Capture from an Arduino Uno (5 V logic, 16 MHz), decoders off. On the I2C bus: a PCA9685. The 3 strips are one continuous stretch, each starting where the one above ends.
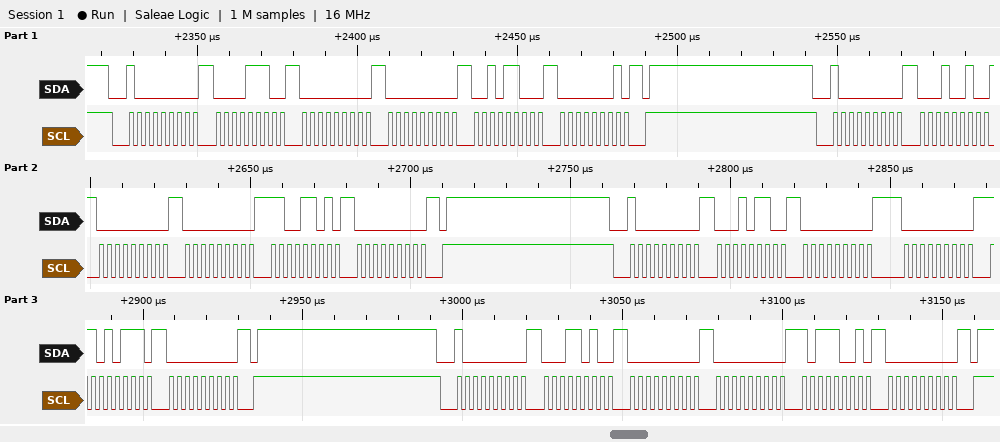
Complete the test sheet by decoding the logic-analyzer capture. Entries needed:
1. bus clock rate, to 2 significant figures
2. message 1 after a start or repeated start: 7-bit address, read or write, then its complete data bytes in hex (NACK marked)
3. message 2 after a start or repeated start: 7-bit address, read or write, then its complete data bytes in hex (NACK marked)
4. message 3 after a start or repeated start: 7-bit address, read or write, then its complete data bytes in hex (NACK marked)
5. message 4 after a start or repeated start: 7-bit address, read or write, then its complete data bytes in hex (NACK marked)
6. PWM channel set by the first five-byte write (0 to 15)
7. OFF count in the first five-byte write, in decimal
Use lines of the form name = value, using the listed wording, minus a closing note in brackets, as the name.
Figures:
bus clock rate, to 2 significant figures = 400 kHz
message 1 after a start or repeated start: 7-bit address, read or write, then its complete data bytes in hex = 0x40 write: 0E 00 00 2C 01
message 2 after a start or repeated start: 7-bit address, read or write, then its complete data bytes in hex = 0x40 write: 12 00 00 CD 00
message 3 after a start or repeated start: 7-bit address, read or write, then its complete data bytes in hex = 0x40 write: 16 00 00 D7 00
message 4 after a start or repeated start: 7-bit address, read or write, then its complete data bytes in hex = 0x40 write: 1A 00 00 B9 00
PWM channel set by the first five-byte write = 2
OFF count in the first five-byte write, in decimal = 300
